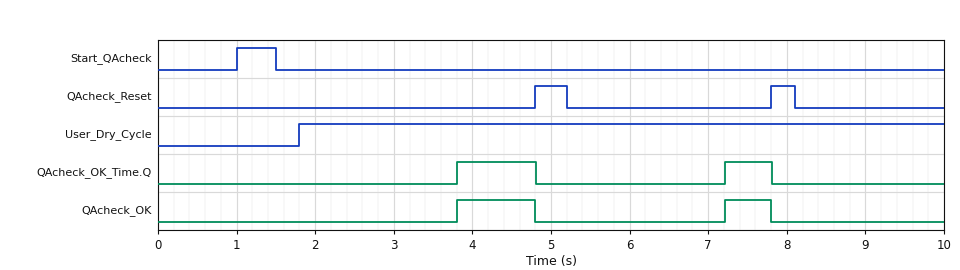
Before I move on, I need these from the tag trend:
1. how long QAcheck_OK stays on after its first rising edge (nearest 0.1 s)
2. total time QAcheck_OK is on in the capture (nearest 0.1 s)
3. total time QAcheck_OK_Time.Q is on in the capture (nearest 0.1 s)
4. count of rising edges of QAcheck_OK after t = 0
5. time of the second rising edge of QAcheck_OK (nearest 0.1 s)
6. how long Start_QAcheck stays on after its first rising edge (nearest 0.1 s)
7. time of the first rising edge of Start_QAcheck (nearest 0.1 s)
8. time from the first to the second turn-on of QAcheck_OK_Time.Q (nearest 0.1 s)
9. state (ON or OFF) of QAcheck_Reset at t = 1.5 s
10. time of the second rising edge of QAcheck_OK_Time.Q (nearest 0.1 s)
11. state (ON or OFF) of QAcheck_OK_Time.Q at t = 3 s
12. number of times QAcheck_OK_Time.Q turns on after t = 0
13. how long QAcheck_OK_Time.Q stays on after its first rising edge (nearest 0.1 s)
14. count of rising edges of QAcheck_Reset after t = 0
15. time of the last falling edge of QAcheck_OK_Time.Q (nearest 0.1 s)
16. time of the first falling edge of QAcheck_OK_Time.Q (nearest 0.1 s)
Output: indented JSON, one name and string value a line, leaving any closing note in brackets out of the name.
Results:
{
  "how long QAcheck_OK stays on after its first rising edge": "1.0 s",
  "total time QAcheck_OK is on in the capture": "1.6 s",
  "total time QAcheck_OK_Time.Q is on in the capture": "1.6 s",
  "count of rising edges of QAcheck_OK after t = 0": "2",
  "time of the second rising edge of QAcheck_OK": "7.2 s",
  "how long Start_QAcheck stays on after its first rising edge": "0.5 s",
  "time of the first rising edge of Start_QAcheck": "1.0 s",
  "time from the first to the second turn-on of QAcheck_OK_Time.Q": "3.4 s",
  "state (ON or OFF) of QAcheck_Reset at t = 1.5 s": "OFF",
  "time of the second rising edge of QAcheck_OK_Time.Q": "7.2 s",
  "state (ON or OFF) of QAcheck_OK_Time.Q at t = 3 s": "OFF",
  "number of times QAcheck_OK_Time.Q turns on after t = 0": "2",
  "how long QAcheck_OK_Time.Q stays on after its first rising edge": "1.0 s",
  "count of rising edges of QAcheck_Reset after t = 0": "2",
  "time of the last falling edge of QAcheck_OK_Time.Q": "7.8 s",
  "time of the first falling edge of QAcheck_OK_Time.Q": "4.8 s"
}
